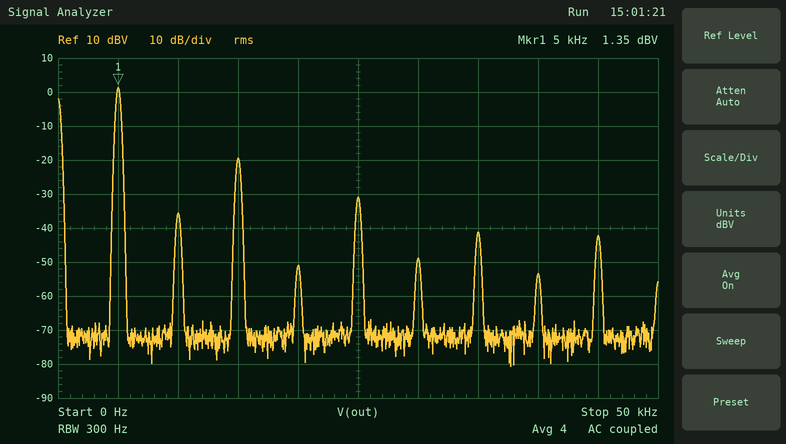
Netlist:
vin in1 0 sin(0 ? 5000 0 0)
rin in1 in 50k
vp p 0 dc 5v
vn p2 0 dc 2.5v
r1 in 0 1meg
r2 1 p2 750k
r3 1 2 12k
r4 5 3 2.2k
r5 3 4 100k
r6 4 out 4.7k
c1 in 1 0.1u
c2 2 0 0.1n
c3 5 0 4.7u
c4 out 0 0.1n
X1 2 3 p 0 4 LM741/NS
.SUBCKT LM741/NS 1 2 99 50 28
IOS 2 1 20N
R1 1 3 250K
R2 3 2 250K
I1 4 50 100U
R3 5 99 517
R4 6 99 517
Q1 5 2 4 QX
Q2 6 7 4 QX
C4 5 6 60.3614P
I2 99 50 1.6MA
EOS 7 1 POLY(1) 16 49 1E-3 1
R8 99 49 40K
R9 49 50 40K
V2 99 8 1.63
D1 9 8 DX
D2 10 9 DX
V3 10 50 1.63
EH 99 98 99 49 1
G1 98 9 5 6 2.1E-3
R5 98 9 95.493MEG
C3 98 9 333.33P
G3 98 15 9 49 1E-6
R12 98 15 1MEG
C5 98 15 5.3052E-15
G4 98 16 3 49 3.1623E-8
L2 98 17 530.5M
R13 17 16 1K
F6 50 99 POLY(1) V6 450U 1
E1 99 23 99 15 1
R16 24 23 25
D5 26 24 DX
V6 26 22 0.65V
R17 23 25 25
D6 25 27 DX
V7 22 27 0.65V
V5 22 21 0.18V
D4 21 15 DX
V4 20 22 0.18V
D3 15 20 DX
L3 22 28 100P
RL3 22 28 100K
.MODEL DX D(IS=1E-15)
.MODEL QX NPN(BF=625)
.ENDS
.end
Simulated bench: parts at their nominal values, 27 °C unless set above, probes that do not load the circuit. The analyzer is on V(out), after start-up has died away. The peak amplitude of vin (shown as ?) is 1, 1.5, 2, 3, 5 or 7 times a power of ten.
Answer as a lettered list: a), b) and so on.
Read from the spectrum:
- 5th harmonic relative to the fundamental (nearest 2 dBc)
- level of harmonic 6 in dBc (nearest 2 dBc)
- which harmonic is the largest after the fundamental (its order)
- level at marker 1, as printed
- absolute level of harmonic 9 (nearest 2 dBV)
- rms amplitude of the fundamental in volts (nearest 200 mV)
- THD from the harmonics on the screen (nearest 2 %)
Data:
a) -32 dBc
b) -50 dBc
c) 3
d) 1.35 dBV
e) -42 dBV
f) 1.2 V
g) 10 %
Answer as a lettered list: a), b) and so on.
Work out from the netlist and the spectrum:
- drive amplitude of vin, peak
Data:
a) 50 mV
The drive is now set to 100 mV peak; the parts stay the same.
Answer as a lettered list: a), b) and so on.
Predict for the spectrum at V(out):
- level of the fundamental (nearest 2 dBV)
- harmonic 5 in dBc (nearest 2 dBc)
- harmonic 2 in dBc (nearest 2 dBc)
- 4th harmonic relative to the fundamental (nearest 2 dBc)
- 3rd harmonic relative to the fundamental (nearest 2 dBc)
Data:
a) 2 dBV
b) -24 dBc
c) -38 dBc
d) -44 dBc
e) -12 dBc
